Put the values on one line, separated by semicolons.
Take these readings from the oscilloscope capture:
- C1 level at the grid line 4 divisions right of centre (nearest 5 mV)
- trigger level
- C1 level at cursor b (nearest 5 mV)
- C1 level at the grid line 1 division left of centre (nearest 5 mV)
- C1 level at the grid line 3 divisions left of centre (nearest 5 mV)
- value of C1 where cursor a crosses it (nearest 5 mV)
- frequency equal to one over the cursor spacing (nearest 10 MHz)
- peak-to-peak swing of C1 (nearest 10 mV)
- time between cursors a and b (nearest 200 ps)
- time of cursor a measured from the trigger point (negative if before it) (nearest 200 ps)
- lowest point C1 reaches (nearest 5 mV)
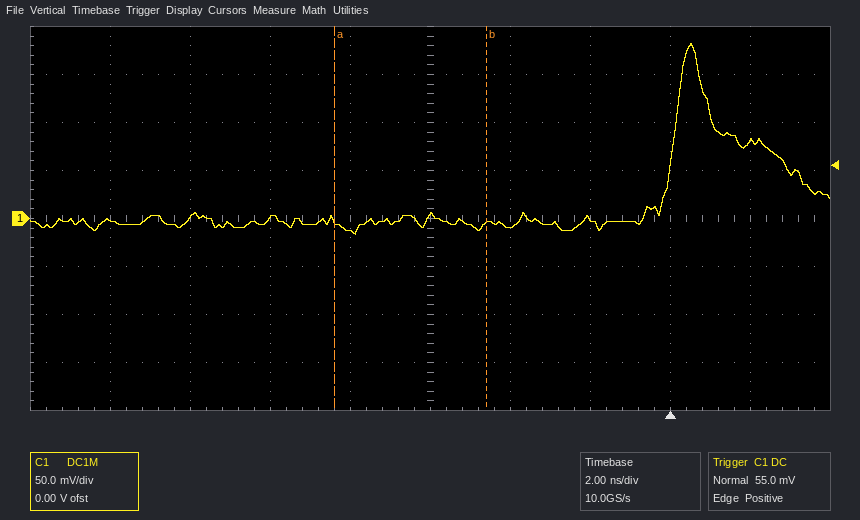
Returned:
80 mV; 55.0 mV; -5 mV; -15 mV; 0 mV; 0 mV; 260 MHz; 200 mV; 3.8 ns; -8.4 ns; -15 mV
